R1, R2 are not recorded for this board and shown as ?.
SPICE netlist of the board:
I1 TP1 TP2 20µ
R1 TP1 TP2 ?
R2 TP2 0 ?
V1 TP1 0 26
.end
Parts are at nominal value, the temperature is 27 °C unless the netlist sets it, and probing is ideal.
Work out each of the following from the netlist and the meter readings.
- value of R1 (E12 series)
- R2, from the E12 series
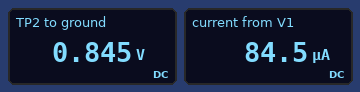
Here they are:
390 kΩ
10 kΩ
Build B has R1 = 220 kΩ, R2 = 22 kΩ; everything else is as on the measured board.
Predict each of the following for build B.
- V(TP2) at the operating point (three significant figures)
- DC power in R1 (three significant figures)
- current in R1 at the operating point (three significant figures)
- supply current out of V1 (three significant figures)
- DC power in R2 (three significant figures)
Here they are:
2.76 V
2.45 mW
106 µA
126 µA
347 µW
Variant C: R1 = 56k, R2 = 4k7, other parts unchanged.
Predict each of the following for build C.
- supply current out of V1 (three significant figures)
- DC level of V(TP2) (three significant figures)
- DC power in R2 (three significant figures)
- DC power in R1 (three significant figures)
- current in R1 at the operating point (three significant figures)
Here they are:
447 µA
2.10 V
938 µW
10.2 mW
427 µA
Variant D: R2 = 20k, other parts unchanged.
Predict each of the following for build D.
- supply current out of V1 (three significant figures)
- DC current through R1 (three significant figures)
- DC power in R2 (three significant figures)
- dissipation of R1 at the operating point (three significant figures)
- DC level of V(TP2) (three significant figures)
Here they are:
82.4 µA
62.4 µA
136 µW
1.52 mW
1.65 V
